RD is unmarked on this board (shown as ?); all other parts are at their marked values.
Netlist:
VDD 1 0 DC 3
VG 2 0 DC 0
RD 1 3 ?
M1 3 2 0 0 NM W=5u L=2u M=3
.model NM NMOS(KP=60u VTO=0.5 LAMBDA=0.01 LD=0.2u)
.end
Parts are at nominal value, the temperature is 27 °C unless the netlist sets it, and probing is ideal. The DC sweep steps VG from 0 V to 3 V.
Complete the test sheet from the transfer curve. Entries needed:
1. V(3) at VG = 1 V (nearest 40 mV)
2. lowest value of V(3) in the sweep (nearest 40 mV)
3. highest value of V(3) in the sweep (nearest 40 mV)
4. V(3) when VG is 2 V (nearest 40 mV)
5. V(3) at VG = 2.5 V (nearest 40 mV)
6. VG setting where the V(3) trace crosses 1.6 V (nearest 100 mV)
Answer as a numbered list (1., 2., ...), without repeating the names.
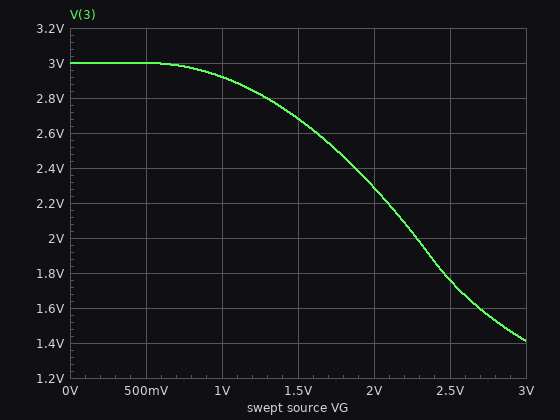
1. 2.92 V
2. 1.40 V
3. 3.00 V
4. 2.28 V
5. 1.76 V
6. 2.7 V
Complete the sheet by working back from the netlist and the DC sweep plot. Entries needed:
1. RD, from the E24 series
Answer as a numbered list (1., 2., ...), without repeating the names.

1. 1.1 kΩ
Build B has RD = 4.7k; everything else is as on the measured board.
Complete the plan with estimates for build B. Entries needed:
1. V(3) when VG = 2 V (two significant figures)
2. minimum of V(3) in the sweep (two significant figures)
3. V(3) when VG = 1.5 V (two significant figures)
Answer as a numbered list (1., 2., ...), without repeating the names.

1. 750 mV
2. 420 mV
3. 1.7 V
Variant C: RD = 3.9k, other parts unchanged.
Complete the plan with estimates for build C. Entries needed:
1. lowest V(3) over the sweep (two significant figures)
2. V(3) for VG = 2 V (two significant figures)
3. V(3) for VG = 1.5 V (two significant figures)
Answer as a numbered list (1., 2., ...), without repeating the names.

1. 500 mV
2. 900 mV
3. 1.9 V
